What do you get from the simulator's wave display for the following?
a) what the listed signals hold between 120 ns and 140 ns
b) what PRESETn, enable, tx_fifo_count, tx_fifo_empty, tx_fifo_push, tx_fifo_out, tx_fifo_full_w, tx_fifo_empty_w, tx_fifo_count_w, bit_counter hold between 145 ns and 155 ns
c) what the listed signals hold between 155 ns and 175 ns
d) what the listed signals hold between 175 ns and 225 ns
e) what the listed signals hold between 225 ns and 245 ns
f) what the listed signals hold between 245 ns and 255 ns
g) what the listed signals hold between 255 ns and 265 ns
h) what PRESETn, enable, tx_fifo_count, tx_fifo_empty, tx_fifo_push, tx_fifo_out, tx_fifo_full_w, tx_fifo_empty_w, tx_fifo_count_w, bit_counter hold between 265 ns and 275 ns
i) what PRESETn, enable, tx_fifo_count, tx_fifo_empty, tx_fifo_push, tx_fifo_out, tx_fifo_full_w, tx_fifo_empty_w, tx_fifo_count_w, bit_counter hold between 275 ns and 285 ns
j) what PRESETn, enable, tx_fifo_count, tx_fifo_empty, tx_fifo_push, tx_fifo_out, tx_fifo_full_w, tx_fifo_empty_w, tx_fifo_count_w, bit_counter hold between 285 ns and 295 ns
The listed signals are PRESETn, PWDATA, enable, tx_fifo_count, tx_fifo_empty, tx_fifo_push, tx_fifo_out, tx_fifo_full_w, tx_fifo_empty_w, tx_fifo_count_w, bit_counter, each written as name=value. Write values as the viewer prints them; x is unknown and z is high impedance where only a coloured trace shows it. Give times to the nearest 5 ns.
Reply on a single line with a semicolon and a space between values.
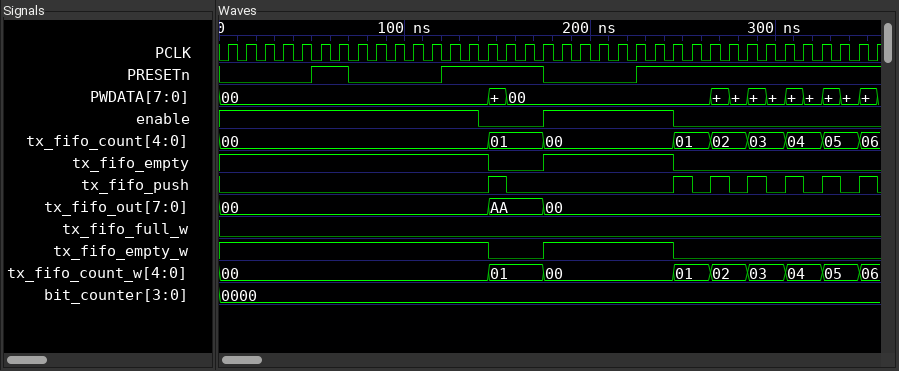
PRESETn=1, PWDATA=00, enable=1, tx_fifo_count=00, tx_fifo_empty=1, tx_fifo_push=0, tx_fifo_out=00, tx_fifo_full_w=0, tx_fifo_empty_w=1, tx_fifo_count_w=00, bit_counter=0000; PRESETn=1, enable=0, tx_fifo_count=01, tx_fifo_empty=0, tx_fifo_push=1, tx_fifo_out=AA, tx_fifo_full_w=0, tx_fifo_empty_w=0, tx_fifo_count_w=01, bit_counter=0000; PRESETn=1, PWDATA=00, enable=0, tx_fifo_count=01, tx_fifo_empty=0, tx_fifo_push=0, tx_fifo_out=AA, tx_fifo_full_w=0, tx_fifo_empty_w=0, tx_fifo_count_w=01, bit_counter=0000; PRESETn=0, PWDATA=00, enable=1, tx_fifo_count=00, tx_fifo_empty=1, tx_fifo_push=0, tx_fifo_out=00, tx_fifo_full_w=0, tx_fifo_empty_w=1, tx_fifo_count_w=00, bit_counter=0000; PRESETn=1, PWDATA=00, enable=1, tx_fifo_count=00, tx_fifo_empty=1, tx_fifo_push=0, tx_fifo_out=00, tx_fifo_full_w=0, tx_fifo_empty_w=1, tx_fifo_count_w=00, bit_counter=0000; PRESETn=1, PWDATA=00, enable=0, tx_fifo_count=01, tx_fifo_empty=0, tx_fifo_push=1, tx_fifo_out=00, tx_fifo_full_w=0, tx_fifo_empty_w=0, tx_fifo_count_w=01, bit_counter=0000; PRESETn=1, PWDATA=00, enable=0, tx_fifo_count=01, tx_fifo_empty=0, tx_fifo_push=0, tx_fifo_out=00, tx_fifo_full_w=0, tx_fifo_empty_w=0, tx_fifo_count_w=01, bit_counter=0000; PRESETn=1, enable=0, tx_fifo_count=02, tx_fifo_empty=0, tx_fifo_push=1, tx_fifo_out=00, tx_fifo_full_w=0, tx_fifo_empty_w=0, tx_fifo_count_w=02, bit_counter=0000; PRESETn=1, enable=0, tx_fifo_count=02, tx_fifo_empty=0, tx_fifo_push=0, tx_fifo_out=00, tx_fifo_full_w=0, tx_fifo_empty_w=0, tx_fifo_count_w=02, bit_counter=0000; PRESETn=1, enable=0, tx_fifo_count=03, tx_fifo_empty=0, tx_fifo_push=1, tx_fifo_out=00, tx_fifo_full_w=0, tx_fifo_empty_w=0, tx_fifo_count_w=03, bit_counter=0000
